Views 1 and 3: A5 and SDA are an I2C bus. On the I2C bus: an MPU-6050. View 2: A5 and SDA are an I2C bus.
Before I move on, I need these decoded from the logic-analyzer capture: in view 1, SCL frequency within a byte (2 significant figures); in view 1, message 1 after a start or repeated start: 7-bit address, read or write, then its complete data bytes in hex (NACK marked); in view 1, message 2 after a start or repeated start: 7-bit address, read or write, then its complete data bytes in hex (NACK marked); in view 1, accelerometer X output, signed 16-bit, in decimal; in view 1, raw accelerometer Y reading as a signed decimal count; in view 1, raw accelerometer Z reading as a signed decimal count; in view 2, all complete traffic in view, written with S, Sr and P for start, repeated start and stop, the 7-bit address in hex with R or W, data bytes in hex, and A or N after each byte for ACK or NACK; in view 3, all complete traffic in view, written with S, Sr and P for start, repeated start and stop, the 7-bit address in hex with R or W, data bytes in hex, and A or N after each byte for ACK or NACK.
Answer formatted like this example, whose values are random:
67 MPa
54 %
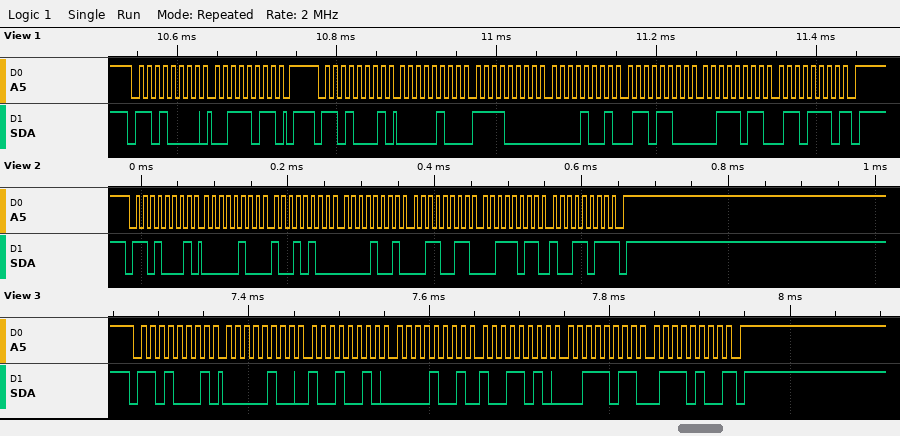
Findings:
100 kHz
0x68 write: 3B
0x68 read: 04 F0 09 6C 3B 6E NACK
1264
2412
15214
S 68R A 04 A 94 A 09 A 33 A 3B A 9B N P
S 68R A 04 A 92 A 09 A 9A A 3B A 74 N P
